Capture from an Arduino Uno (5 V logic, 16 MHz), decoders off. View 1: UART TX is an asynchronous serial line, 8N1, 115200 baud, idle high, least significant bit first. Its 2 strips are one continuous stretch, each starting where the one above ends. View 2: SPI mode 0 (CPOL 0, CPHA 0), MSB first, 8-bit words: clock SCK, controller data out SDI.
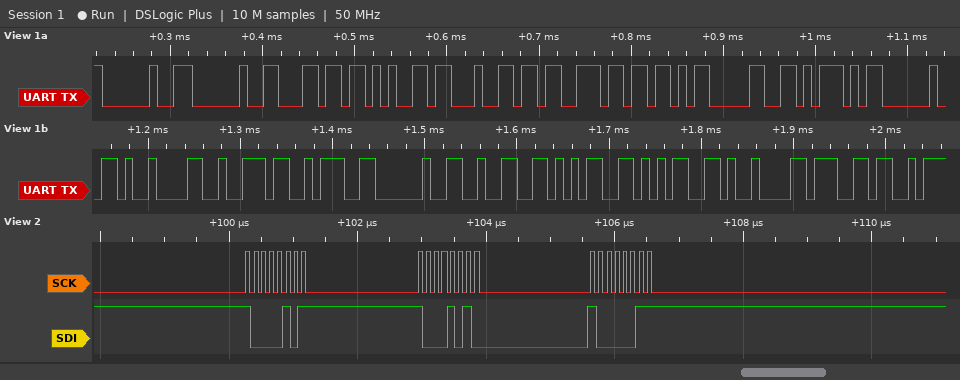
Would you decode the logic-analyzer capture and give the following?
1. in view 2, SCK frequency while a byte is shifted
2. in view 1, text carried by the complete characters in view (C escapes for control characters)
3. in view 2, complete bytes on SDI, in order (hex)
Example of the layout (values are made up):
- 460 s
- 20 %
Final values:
- 8 MHz
- "  leds[0] \tr: 255\tg"
- 85 8A 83
